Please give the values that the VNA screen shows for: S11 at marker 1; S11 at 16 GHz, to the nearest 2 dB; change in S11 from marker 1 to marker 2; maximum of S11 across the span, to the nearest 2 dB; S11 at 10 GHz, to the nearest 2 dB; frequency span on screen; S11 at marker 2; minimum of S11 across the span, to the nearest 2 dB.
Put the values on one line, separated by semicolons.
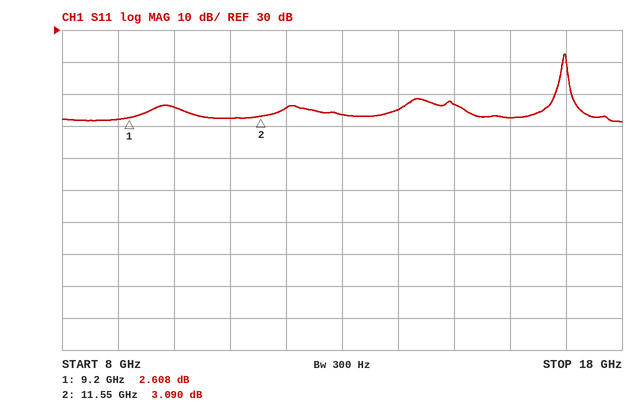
2.608 dB; 2 dB; 0.482 dB; 22 dB; 6 dB; 10 GHz; 3.090 dB; 2 dB
